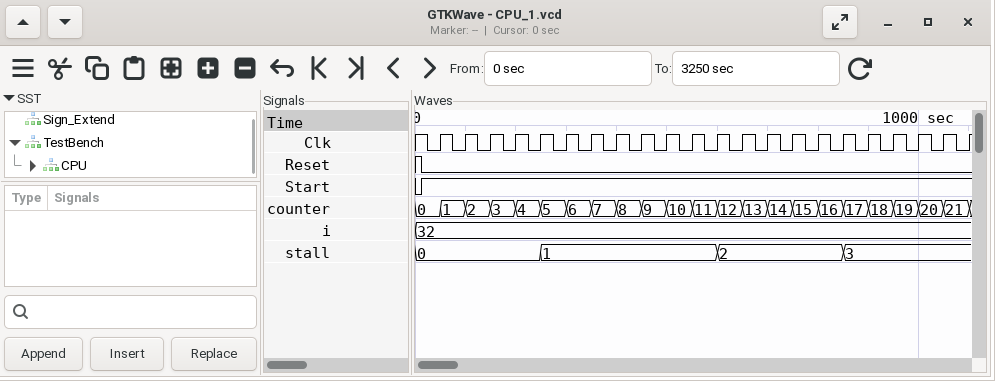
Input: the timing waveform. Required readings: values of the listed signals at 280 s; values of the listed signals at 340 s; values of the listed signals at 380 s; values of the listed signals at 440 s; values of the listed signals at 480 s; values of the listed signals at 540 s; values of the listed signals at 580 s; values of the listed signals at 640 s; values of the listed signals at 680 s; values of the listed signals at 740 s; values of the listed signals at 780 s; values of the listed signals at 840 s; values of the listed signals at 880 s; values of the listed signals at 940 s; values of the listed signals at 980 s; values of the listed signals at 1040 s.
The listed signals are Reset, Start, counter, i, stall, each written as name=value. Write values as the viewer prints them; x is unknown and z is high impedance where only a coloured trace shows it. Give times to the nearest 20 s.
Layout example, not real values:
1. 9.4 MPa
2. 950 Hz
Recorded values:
1. Reset=0, Start=1, counter=5, i=32, stall=1
2. Reset=0, Start=1, counter=6, i=32, stall=1
3. Reset=0, Start=1, counter=7, i=32, stall=1
4. Reset=0, Start=1, counter=8, i=32, stall=1
5. Reset=0, Start=1, counter=9, i=32, stall=1
6. Reset=0, Start=1, counter=10, i=32, stall=1
7. Reset=0, Start=1, counter=11, i=32, stall=1
8. Reset=0, Start=1, counter=12, i=32, stall=2
9. Reset=0, Start=1, counter=13, i=32, stall=2
10. Reset=0, Start=1, counter=14, i=32, stall=2
11. Reset=0, Start=1, counter=15, i=32, stall=2
12. Reset=0, Start=1, counter=16, i=32, stall=2
13. Reset=0, Start=1, counter=17, i=32, stall=3
14. Reset=0, Start=1, counter=18, i=32, stall=3
15. Reset=0, Start=1, counter=19, i=32, stall=3
16. Reset=0, Start=1, counter=20, i=32, stall=3
